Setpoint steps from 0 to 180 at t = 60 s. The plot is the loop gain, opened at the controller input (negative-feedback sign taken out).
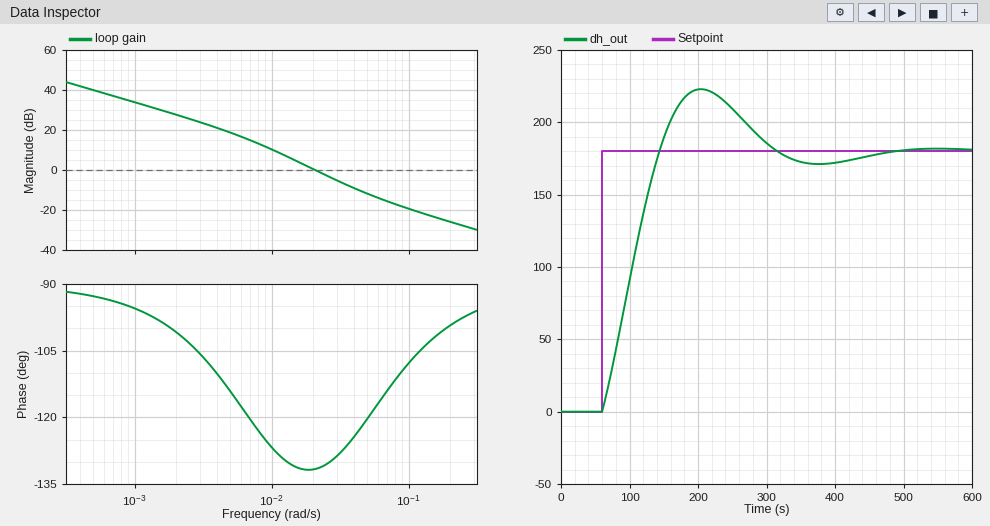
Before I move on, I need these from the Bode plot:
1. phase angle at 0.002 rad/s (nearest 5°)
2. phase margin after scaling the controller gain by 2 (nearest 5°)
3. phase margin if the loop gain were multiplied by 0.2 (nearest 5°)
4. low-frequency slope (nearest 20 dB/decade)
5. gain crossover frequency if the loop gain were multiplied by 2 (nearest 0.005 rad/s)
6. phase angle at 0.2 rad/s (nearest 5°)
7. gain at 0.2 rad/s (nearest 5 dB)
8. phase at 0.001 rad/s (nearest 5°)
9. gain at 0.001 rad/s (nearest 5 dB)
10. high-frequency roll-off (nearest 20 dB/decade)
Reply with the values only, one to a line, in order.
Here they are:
-100°
50°
60°
-20 dB/decade
0.030 rad/s
-100°
-25 dB
-95°
35 dB
-20 dB/decade
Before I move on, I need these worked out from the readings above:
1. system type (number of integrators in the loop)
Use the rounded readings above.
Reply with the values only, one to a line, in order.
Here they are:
1
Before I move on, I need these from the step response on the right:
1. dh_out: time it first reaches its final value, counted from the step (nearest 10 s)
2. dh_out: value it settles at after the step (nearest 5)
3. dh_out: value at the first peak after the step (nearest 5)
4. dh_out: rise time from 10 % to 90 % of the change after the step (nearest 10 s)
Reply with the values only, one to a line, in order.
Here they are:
80 s
180
225
60 s
